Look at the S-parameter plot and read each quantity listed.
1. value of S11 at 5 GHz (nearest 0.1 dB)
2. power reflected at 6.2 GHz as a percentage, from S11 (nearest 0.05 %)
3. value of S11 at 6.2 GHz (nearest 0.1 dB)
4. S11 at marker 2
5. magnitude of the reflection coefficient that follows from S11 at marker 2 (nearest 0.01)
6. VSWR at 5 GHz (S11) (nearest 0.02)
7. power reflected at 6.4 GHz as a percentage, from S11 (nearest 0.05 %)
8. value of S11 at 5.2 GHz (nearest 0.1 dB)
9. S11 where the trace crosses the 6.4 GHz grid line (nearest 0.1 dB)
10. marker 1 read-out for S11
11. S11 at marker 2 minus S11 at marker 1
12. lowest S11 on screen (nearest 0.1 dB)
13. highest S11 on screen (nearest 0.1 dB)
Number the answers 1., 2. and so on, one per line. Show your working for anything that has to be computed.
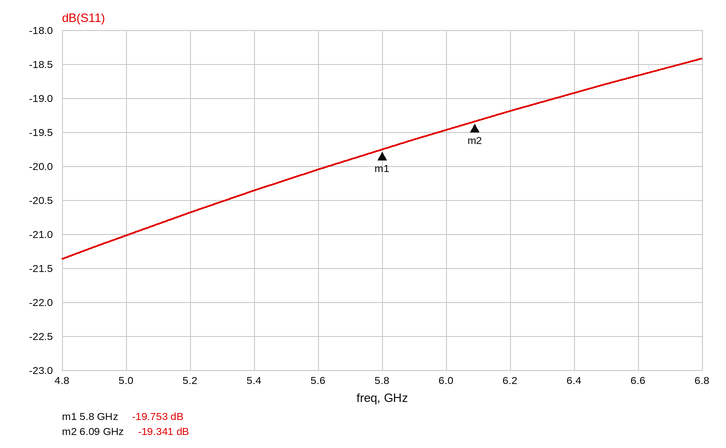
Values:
1. -21.0 dB
2. 10^(-19.2/10) ≈ 1.20 %
3. -19.2 dB
4. -19.341 dB
5. 10^(-19.341/20) ≈ 0.11
6. |Γ| = 10^(-21/20) = 0.0891; VSWR = (1 + 0.0891)/(1 − 0.0891) ≈ 1.20
7. 10^(-18.9/10) ≈ 1.29 %, so 1.30 % to the nearest 0.05 %
8. -20.7 dB
9. -18.9 dB
10. -19.753 dB
11. -19.341 − (-19.753) = 0.412 dB
12. -21.4 dB
13. -18.4 dB
